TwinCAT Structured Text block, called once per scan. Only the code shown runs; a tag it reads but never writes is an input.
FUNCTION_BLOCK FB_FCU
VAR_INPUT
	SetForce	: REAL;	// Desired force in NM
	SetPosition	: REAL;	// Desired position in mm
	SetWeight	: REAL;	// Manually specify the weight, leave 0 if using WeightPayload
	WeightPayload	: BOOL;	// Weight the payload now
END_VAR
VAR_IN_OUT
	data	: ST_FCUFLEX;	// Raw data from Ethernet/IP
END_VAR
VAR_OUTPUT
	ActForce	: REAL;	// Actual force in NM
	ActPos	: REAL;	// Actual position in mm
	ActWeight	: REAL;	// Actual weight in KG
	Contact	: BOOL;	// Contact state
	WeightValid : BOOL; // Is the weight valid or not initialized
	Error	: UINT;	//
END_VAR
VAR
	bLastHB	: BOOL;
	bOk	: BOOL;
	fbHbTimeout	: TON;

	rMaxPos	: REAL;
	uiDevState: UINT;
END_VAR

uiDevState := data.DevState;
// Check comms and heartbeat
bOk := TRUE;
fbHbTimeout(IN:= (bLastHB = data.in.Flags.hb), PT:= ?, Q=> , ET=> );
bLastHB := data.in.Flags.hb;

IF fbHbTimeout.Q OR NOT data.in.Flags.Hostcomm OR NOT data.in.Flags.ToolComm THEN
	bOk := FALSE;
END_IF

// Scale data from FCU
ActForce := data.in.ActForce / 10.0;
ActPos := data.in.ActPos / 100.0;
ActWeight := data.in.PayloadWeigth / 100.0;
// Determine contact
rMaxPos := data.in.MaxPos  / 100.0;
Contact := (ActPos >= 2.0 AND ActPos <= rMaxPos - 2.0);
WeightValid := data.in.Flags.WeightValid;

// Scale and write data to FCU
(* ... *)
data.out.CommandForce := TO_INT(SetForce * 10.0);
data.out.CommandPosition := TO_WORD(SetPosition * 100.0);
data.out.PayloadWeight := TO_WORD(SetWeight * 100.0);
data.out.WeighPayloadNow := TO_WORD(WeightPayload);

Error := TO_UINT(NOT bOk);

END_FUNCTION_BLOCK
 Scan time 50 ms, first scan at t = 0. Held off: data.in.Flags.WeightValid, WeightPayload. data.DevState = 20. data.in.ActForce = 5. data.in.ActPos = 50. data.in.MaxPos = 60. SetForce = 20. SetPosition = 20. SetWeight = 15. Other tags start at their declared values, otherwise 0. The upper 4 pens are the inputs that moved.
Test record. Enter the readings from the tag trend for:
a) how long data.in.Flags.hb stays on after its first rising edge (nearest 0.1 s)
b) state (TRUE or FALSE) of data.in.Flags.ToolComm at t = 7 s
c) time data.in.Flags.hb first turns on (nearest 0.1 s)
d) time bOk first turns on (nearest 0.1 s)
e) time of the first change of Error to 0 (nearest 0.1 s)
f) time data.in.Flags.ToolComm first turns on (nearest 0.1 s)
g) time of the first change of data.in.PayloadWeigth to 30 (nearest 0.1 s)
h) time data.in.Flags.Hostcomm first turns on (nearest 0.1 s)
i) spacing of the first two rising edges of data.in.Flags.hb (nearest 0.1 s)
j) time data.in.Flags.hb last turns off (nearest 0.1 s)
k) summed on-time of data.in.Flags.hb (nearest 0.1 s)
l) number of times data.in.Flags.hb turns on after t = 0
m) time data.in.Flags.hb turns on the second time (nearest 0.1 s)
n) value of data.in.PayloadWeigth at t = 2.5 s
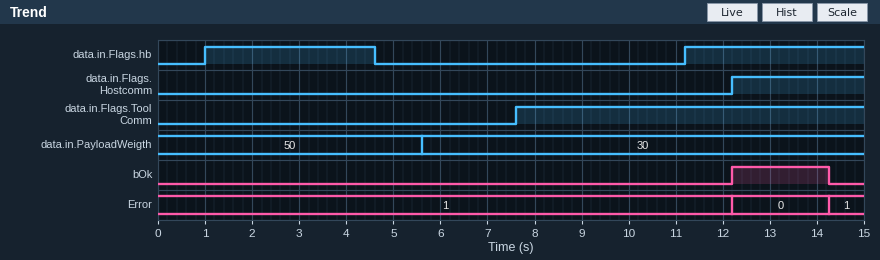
3.6 s
FALSE
1.0 s
12.2 s
12.2 s
7.6 s
5.6 s
12.2 s
10.2 s
4.6 s
7.4 s
2
11.2 s
50
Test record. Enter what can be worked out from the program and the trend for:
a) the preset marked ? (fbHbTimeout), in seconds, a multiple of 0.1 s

3.0 s
